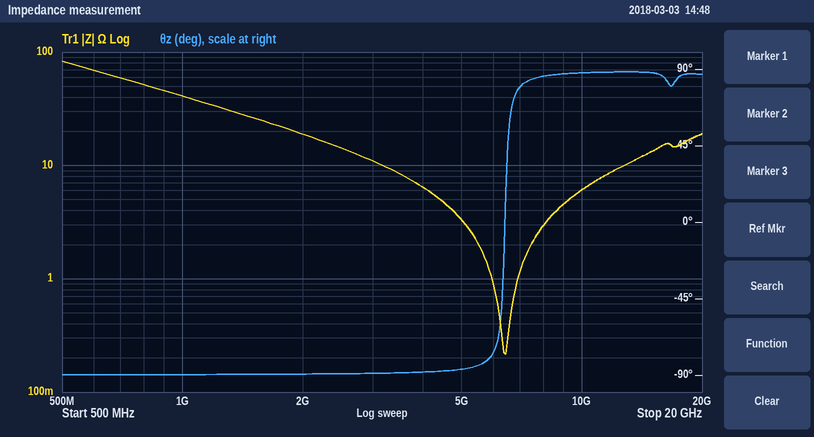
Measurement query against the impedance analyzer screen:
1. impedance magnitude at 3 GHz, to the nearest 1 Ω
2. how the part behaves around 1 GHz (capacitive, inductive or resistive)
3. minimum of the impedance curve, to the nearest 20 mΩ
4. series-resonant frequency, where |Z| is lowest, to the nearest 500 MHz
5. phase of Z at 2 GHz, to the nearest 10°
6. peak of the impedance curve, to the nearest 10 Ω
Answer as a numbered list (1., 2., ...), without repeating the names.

1. 11 Ω
2. capacitive
3. 220 mΩ
4. 6.5 GHz
5. -90°
6. 80 Ω
